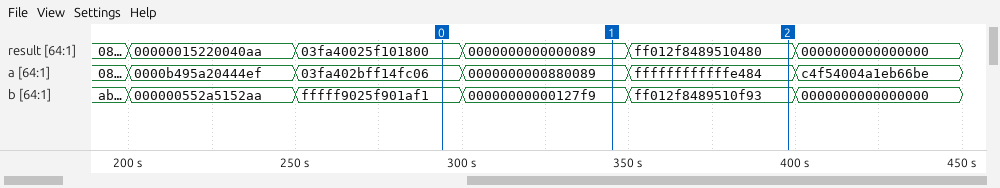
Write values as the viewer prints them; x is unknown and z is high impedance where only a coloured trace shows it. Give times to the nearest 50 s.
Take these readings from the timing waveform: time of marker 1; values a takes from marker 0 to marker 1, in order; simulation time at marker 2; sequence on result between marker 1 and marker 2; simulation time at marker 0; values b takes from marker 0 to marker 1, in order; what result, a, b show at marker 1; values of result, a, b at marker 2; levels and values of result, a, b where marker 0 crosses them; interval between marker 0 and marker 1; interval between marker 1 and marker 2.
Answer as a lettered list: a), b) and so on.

a) 350 s
b) 03fa402bff14fc06, 0000000000880089
c) 400 s
d) 0000000000000089, ff012f8489510480
e) 300 s
f) fffff9025f901af1, 00000000000127f9
g) result=0000000000000089, a=0000000000880089, b=00000000000127f9
h) result=ff012f8489510480, a=ffffffffffffe484, b=ff012f8489510f93
i) result=03fa40025f101800, a=03fa402bff14fc06, b=fffff9025f901af1
j) 50 s
k) 50 s
